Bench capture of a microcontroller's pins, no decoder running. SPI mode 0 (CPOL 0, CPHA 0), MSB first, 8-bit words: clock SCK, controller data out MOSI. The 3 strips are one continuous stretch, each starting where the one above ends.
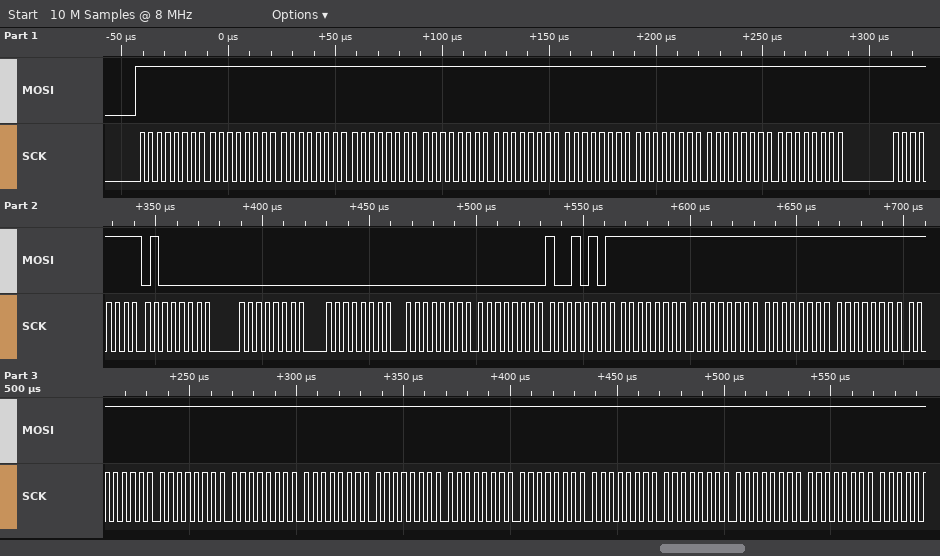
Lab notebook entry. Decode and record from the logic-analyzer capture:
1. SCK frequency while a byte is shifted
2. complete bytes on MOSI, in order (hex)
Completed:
250 kHz
FF FF FF FF FF FF FF FF FF FF FF 40 00 00 00 00 95 FF FF FF FF FF FF FF FF FF FF FF FF FF FF FF
